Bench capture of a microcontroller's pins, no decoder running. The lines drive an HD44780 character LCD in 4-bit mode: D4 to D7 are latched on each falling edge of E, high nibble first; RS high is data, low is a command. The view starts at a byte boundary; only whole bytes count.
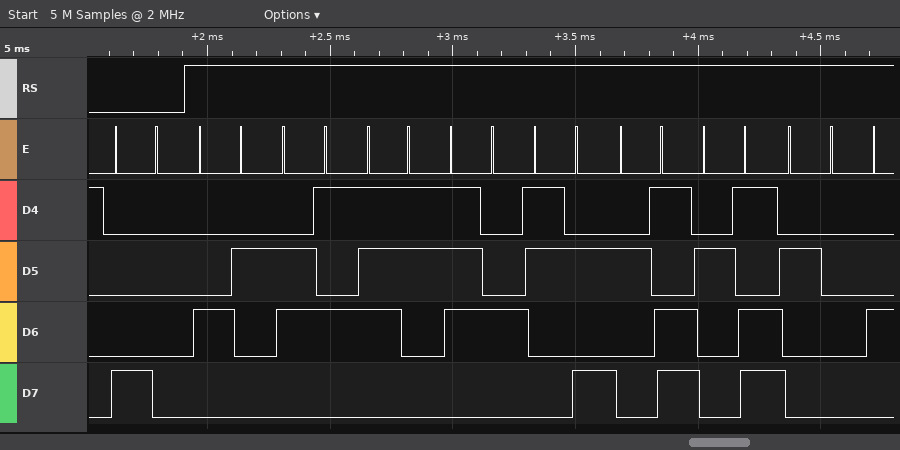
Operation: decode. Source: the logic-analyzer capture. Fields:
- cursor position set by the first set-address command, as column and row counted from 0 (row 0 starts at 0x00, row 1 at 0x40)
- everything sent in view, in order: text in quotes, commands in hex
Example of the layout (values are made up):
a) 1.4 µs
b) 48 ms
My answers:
a) column 0, row 0
b) 0x80 "Best:-- "
